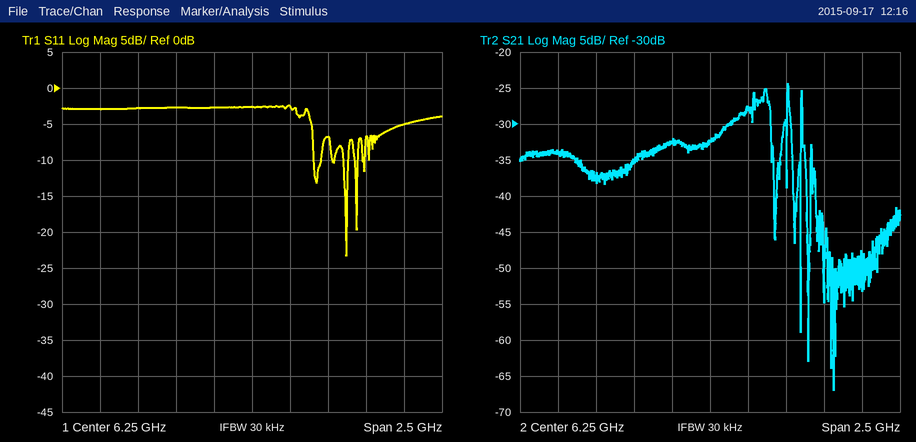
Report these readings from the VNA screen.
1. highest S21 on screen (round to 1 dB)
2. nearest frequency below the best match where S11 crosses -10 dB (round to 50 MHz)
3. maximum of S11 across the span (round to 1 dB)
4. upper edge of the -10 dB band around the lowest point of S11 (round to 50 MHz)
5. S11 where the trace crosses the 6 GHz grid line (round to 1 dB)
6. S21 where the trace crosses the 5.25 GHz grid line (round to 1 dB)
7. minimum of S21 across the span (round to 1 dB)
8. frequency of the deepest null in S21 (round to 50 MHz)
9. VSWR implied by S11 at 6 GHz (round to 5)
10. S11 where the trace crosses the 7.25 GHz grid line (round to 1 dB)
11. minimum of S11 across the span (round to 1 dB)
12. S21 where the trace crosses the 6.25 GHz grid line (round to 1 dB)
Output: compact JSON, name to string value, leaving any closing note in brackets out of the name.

{"highest S21 on screen": "-24 dB", "nearest frequency below the best match where S11 crosses -10 dB": "6.85 GHz", "maximum of S11 across the span": "-2 dB", "upper edge of the -10 dB band around the lowest point of S11": "6.90 GHz", "S11 where the trace crosses the 6 GHz grid line": "-3 dB", "S21 where the trace crosses the 5.25 GHz grid line": "-34 dB", "minimum of S21 across the span": "-67 dB", "frequency of the deepest null in S21": "7.05 GHz", "VSWR implied by S11 at 6 GHz": "5", "S11 where the trace crosses the 7.25 GHz grid line": "-5 dB", "minimum of S11 across the span": "-23 dB", "S21 where the trace crosses the 6.25 GHz grid line": "-32 dB"}
